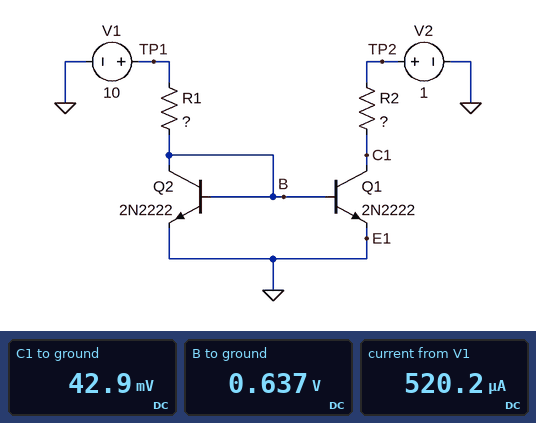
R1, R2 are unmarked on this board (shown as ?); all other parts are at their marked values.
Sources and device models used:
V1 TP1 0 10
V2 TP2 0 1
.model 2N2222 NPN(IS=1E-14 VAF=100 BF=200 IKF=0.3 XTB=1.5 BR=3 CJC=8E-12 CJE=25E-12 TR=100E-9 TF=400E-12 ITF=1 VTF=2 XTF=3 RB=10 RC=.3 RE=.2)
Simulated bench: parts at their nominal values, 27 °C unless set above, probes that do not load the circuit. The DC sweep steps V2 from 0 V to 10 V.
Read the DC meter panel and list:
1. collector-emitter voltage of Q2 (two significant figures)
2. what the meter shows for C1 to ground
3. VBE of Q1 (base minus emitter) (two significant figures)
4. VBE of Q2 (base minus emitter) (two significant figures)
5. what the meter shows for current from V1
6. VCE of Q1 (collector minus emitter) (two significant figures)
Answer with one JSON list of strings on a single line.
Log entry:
["640 mV", "42.9 mV", "640 mV", "640 mV", "520.2 µA", "43 mV"]
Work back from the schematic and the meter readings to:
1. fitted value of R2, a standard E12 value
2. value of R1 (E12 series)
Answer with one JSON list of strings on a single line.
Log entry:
["2.7 kΩ", "18 kΩ"]
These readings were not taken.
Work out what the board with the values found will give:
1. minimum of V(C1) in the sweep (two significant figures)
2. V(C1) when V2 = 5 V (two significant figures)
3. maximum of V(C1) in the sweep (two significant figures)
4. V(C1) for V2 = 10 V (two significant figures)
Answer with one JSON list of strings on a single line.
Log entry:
["7.3 mV", "3.6 V", "8.5 V", "8.5 V"]
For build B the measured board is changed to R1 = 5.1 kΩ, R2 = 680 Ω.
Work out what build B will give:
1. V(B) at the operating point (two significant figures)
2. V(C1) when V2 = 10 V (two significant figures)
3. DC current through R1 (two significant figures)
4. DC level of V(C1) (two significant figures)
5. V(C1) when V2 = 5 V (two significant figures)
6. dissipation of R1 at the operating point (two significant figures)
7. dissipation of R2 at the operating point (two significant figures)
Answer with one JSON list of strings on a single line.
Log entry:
["670 mV", "8.7 V", "1.8 mA", "54 mV", "3.7 V", "17 mW", "1.3 mW"]
